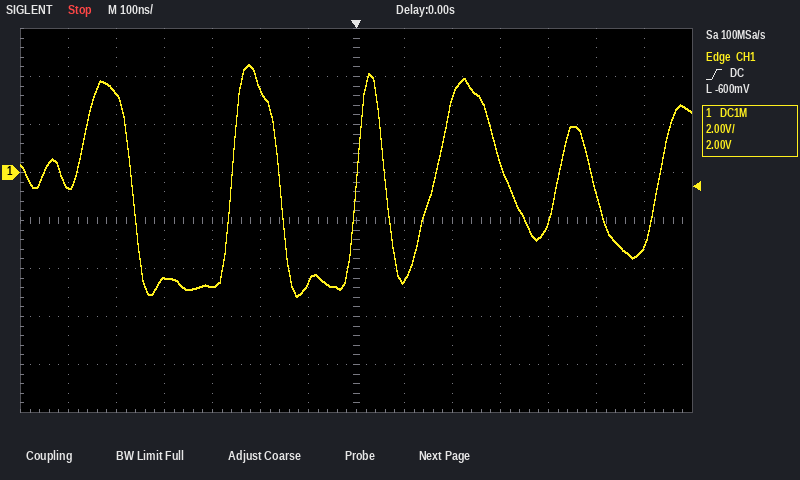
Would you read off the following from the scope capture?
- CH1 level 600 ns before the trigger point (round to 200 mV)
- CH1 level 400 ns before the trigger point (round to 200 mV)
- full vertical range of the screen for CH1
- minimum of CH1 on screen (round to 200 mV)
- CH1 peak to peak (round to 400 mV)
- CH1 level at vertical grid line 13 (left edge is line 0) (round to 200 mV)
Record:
-600 mV
-4.4 V
16 V
-5.2 V
9.6 V
-3.0 V
